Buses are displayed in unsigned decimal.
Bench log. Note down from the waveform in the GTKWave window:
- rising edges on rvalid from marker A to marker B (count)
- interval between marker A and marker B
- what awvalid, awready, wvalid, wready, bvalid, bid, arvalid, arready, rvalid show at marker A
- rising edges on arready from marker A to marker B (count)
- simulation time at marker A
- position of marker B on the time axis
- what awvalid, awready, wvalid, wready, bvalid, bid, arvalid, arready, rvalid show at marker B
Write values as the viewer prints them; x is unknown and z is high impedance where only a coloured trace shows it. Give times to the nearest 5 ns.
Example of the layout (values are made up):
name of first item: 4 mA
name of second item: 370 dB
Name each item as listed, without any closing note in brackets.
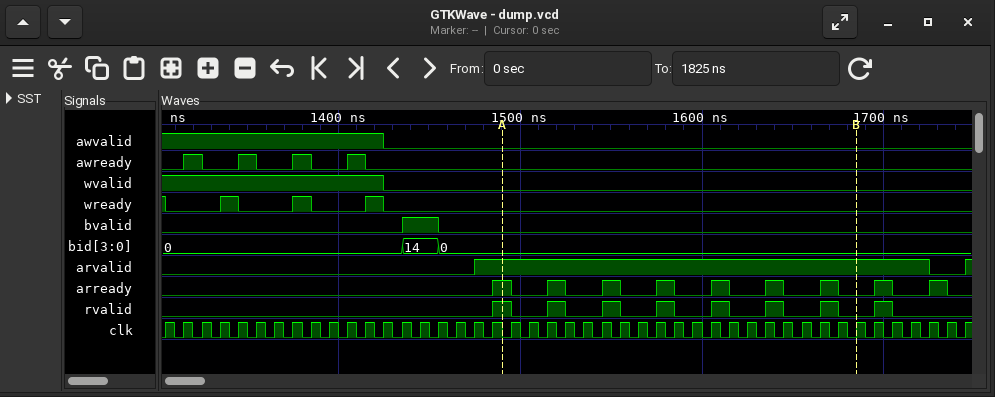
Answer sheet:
rising edges on rvalid from marker A to marker B: 6
interval between marker A and marker B: 195 ns
what awvalid, awready, wvalid, wready, bvalid, bid, arvalid, arready, rvalid show at marker A: awvalid=0, awready=0, wvalid=0, wready=0, bvalid=0, bid=0, arvalid=1, arready=1, rvalid=1
rising edges on arready from marker A to marker B: 6
simulation time at marker A: 1490 ns
position of marker B on the time axis: 1685 ns
what awvalid, awready, wvalid, wready, bvalid, bid, arvalid, arready, rvalid show at marker B: awvalid=0, awready=0, wvalid=0, wready=0, bvalid=0, bid=0, arvalid=1, arready=0, rvalid=0
